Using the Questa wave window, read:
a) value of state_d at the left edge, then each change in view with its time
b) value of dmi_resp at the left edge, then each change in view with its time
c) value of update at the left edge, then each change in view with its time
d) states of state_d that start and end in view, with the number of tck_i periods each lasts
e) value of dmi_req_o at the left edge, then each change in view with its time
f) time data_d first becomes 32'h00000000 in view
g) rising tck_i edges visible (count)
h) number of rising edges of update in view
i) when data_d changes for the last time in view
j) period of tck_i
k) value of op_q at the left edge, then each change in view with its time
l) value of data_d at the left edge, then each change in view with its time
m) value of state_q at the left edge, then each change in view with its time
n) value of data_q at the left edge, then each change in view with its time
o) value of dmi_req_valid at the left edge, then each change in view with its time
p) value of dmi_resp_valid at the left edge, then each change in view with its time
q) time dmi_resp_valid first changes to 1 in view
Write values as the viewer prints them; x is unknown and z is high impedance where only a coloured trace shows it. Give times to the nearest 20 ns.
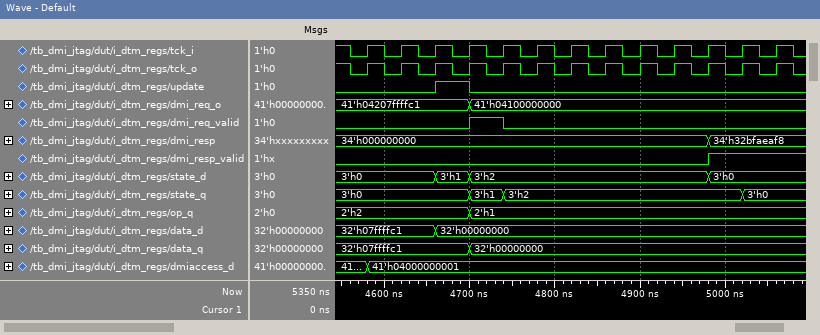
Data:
3'h0, 3'h1 at 4660 ns, 3'h2 at 4700 ns, 3'h0 at 4980 ns
34'h000000000, 34'h32bfaeaf8 at 4980 ns
0, 1 at 4660 ns, 0 at 4700 ns
3'h1: 1, 3'h2: 7
41'h04207ffffc1, 41'h04100000000 at 4700 ns
4660 ns
13
1
4660 ns
40 ns
2'h2, 2'h1 at 4700 ns
32'h07ffffc1, 32'h00000000 at 4660 ns
3'h0, 3'h1 at 4700 ns, 3'h2 at 4740 ns, 3'h0 at 5020 ns
32'h07ffffc1, 32'h00000000 at 4700 ns
0, 1 at 4700 ns, 0 at 4740 ns
0, 1 at 4980 ns
4980 ns
